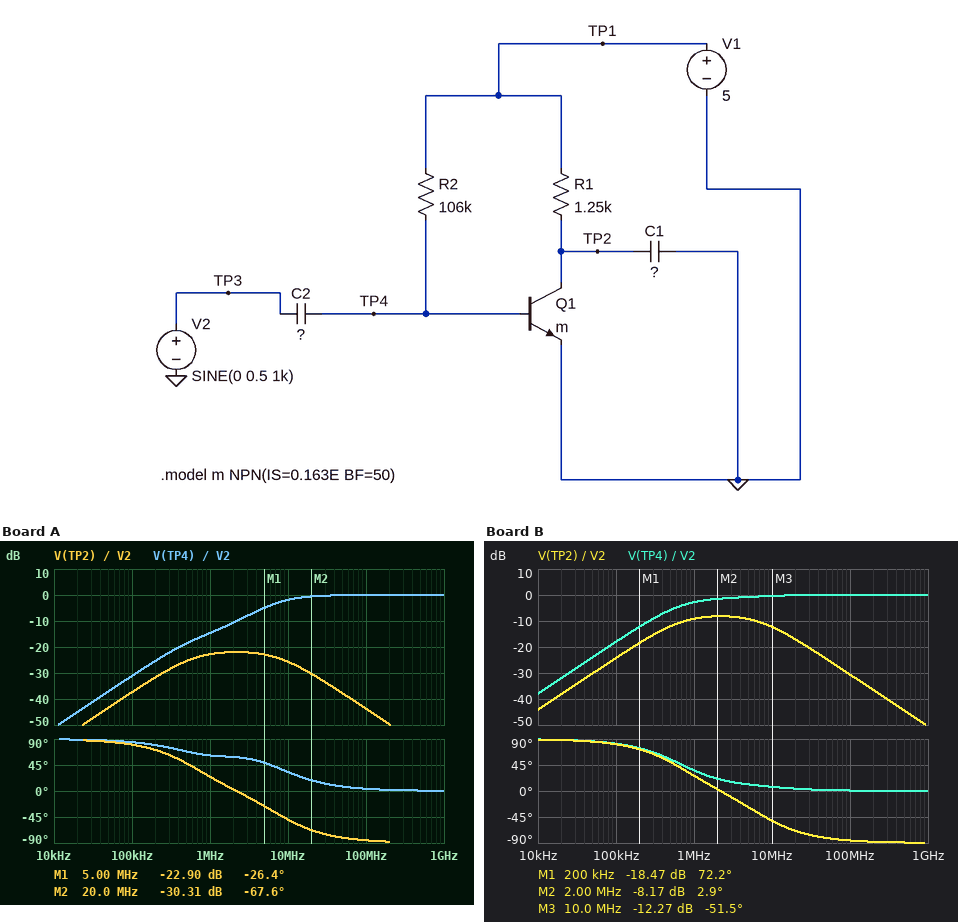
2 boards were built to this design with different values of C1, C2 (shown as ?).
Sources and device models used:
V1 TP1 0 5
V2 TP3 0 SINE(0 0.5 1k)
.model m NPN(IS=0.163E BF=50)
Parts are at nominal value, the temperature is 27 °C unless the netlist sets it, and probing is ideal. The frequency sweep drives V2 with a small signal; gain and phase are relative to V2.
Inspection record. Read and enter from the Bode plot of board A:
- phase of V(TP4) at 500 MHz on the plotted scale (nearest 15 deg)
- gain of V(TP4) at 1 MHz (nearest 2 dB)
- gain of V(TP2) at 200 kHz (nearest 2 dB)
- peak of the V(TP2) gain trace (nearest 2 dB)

0 deg
-14 dB
-32 dB
-22 dB
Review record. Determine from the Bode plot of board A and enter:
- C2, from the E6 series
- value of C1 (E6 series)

150 nF
1.5 µF
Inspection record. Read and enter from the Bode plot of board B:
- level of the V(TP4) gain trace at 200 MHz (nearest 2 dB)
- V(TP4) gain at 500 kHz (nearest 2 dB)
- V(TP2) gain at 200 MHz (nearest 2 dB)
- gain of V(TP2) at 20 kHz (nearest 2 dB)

0 dB
-6 dB
-36 dB
-38 dB
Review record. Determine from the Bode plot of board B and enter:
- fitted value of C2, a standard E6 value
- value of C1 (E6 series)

680 nF
330 nF
